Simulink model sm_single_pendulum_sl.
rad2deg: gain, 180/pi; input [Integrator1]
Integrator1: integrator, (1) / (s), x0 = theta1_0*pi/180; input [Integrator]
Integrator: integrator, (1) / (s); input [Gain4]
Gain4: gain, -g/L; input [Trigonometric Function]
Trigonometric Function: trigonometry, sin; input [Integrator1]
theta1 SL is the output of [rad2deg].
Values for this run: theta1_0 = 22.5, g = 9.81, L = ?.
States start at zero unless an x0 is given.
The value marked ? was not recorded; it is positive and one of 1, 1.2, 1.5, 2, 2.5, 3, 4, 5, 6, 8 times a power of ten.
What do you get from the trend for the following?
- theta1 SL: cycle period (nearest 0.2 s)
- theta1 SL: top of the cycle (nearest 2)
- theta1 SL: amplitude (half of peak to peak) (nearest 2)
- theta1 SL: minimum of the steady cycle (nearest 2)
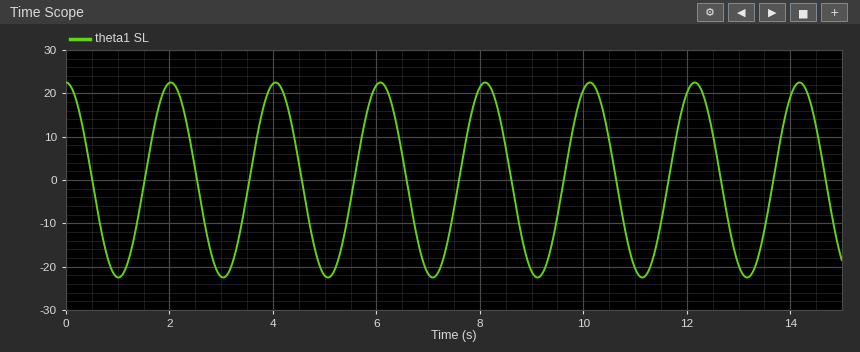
2.0 s
22
22
-22
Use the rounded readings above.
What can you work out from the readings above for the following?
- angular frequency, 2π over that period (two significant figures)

3.1 rad/s
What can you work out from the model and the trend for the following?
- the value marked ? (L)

1
